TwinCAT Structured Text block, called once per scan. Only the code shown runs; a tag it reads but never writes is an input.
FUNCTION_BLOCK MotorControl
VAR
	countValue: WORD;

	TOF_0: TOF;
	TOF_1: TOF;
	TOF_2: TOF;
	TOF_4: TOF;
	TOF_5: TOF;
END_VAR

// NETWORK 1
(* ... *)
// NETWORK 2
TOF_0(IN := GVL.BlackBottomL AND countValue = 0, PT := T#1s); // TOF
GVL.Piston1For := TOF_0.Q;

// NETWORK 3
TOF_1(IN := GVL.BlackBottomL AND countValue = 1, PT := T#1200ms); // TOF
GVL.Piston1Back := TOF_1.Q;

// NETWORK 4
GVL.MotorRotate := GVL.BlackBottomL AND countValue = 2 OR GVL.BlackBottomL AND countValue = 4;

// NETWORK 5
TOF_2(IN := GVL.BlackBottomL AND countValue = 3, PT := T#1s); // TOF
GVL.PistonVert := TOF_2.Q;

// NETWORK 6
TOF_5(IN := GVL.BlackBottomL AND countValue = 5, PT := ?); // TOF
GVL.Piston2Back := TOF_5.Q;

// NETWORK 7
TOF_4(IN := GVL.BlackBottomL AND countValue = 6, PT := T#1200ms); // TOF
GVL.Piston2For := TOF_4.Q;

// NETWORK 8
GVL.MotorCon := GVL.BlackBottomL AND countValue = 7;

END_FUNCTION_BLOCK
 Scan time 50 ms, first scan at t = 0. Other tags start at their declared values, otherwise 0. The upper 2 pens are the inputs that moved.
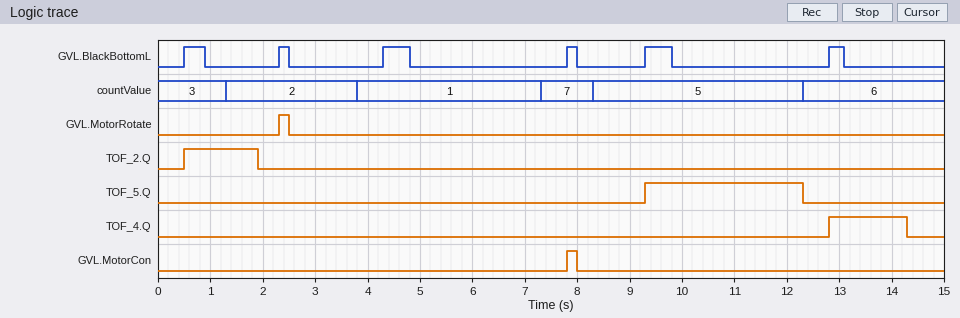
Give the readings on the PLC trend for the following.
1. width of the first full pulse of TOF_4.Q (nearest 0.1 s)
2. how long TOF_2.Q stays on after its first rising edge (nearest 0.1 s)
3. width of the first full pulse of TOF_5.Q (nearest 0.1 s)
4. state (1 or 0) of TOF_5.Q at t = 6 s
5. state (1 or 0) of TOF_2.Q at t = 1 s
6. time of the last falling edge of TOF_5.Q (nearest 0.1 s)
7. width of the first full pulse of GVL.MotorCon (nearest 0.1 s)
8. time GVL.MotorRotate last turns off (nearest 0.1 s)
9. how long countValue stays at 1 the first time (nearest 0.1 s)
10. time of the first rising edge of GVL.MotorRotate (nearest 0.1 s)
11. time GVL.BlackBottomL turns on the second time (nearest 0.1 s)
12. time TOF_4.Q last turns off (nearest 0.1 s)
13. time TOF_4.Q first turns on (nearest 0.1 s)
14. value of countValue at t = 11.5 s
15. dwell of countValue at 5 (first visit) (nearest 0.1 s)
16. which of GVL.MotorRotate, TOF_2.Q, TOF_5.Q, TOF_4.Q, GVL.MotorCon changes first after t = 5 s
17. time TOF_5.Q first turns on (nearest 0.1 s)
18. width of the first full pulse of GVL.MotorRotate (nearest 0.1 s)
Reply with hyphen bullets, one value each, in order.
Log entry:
- 1.5 s
- 1.4 s
- 3.0 s
- 0
- 1
- 12.3 s
- 0.2 s
- 2.5 s
- 3.5 s
- 2.3 s
- 2.3 s
- 14.3 s
- 12.8 s
- 5
- 4.0 s
- GVL.MotorCon
- 9.3 s
- 0.2 s
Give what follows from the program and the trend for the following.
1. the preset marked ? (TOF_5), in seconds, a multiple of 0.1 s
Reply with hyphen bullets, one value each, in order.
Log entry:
- 2.5 s
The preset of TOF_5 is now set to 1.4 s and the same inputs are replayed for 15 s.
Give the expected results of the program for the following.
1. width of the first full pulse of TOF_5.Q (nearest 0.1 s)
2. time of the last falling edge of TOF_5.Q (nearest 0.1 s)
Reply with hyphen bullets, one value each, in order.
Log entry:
- 1.9 s
- 11.2 s
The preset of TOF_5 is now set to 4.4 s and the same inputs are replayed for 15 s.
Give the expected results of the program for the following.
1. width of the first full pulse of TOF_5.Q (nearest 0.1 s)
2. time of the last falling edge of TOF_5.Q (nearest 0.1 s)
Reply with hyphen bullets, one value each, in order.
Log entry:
- 4.9 s
- 14.2 s
